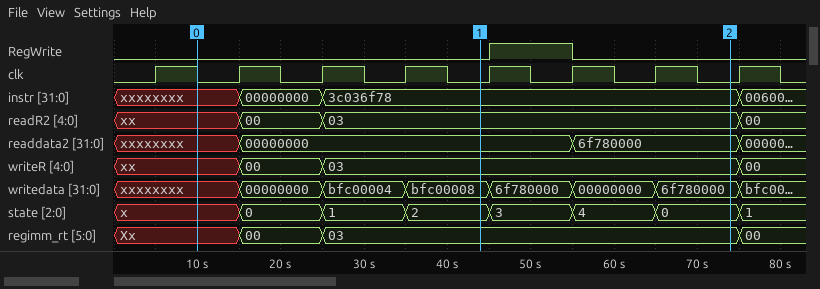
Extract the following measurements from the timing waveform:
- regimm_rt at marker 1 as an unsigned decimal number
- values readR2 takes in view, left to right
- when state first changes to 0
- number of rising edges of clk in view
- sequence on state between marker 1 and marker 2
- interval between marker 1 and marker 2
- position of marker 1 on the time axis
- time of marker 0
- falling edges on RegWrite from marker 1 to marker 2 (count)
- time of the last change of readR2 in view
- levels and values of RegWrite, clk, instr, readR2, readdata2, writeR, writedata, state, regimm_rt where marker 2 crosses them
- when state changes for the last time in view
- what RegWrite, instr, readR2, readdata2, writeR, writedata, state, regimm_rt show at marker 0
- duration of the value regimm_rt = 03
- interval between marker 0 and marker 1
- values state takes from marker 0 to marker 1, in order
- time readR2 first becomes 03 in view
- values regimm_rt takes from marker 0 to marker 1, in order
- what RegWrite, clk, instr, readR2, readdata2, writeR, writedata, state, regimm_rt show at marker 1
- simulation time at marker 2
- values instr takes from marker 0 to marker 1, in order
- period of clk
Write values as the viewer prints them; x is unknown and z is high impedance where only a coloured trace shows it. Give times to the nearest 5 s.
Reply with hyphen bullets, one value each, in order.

- 3
- xx, 00, 03, 00
- 15 s
- 8
- 2, 3, 4, 0
- 30 s
- 45 s
- 10 s
- 1
- 75 s
- RegWrite=0, clk=0, instr=3c036f78, readR2=03, readdata2=6f780000, writeR=03, writedata=6f780000, state=0, regimm_rt=03
- 75 s
- RegWrite=0, instr=xxxxxxxx, readR2=xx, readdata2=xxxxxxxx, writeR=xx, writedata=xxxxxxxx, state=x, regimm_rt=Xx
- 50 s
- 35 s
- x, 0, 1, 2
- 25 s
- Xx, 00, 03
- RegWrite=0, clk=0, instr=3c036f78, readR2=03, readdata2=00000000, writeR=03, writedata=bfc00008, state=2, regimm_rt=03
- 75 s
- xxxxxxxx, 00000000, 3c036f78
- 10 s
